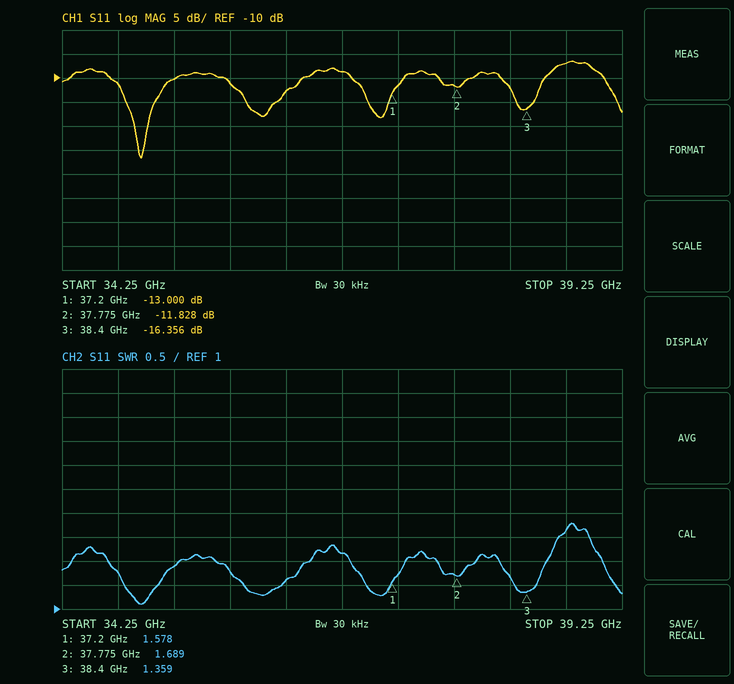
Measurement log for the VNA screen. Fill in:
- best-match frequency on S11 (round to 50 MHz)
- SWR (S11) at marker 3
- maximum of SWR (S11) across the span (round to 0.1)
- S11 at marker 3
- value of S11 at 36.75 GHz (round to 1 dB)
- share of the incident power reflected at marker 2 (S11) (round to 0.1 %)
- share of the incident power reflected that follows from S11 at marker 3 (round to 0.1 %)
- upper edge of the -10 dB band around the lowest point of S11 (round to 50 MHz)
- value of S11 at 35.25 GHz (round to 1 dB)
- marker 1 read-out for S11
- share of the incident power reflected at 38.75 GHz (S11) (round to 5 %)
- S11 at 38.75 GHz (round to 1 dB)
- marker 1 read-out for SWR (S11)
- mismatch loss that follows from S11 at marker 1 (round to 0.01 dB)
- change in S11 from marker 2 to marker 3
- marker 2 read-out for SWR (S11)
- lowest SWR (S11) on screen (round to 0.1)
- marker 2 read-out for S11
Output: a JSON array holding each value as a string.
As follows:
["34.95 GHz", "1.359", "2.8", "-16.356 dB", "-9 dB", "6.6 %", "2.3 %", "35.25 GHz", "-10 dB", "-13.000 dB", "20 %", "-7 dB", "1.578", "0.22 dB", "-4.528 dB", "1.689", "1.1", "-11.828 dB"]
